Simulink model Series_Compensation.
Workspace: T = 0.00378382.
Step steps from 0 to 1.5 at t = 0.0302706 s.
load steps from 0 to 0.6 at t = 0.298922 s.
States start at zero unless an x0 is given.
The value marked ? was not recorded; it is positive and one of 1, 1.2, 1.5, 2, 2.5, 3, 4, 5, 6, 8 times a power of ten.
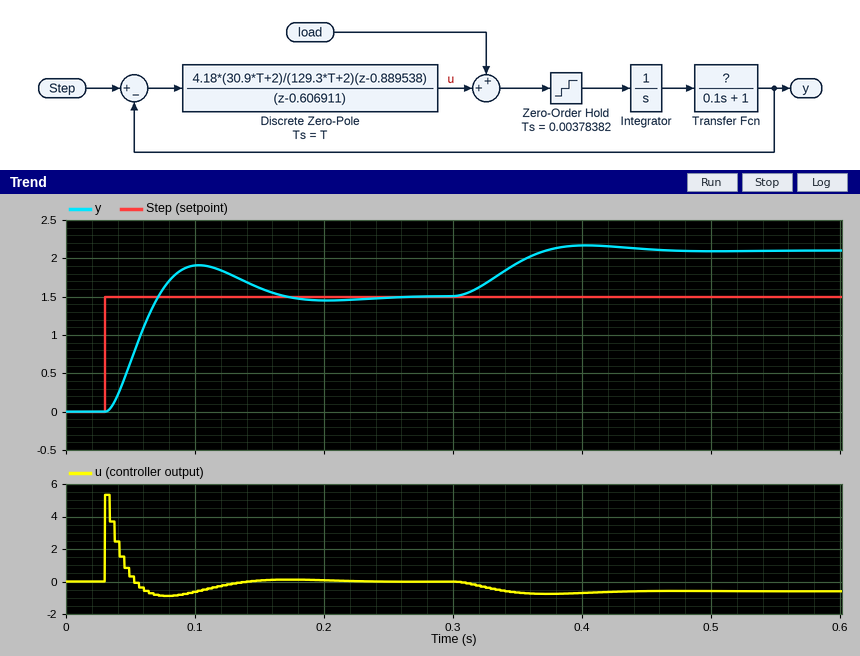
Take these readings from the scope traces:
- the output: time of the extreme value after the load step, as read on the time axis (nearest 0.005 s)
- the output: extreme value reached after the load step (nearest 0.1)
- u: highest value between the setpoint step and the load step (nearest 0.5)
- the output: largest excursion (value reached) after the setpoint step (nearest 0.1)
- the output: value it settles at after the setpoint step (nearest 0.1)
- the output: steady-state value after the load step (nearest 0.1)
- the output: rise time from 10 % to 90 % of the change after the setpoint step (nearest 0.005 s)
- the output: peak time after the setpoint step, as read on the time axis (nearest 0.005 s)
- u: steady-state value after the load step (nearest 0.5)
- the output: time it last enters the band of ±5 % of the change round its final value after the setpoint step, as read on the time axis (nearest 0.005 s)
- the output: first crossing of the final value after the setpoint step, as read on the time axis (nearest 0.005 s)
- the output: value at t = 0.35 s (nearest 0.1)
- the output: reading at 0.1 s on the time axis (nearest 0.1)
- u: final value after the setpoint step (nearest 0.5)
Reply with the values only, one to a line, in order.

0.405 s
2.2
5.5
1.9
1.5
2.1
0.030 s
0.105 s
-0.5
0.155 s
0.070 s
1.9
1.9
0.0
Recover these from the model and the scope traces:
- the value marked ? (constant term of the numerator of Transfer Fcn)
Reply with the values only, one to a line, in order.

100
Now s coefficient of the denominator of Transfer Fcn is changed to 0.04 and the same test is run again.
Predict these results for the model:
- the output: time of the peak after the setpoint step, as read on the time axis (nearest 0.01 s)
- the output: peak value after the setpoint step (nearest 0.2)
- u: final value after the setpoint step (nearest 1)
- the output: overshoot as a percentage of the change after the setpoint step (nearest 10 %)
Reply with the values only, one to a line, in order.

0.07 s
1.8
0
20 %
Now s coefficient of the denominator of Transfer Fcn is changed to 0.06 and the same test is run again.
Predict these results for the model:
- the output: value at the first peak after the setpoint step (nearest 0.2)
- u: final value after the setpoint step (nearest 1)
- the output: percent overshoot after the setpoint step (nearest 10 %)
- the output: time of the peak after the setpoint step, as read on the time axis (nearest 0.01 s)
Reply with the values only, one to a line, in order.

1.8
0
20 %
0.08 s
